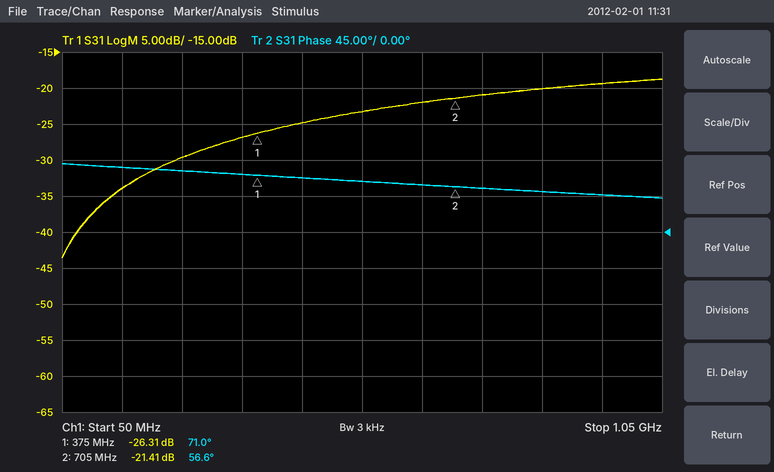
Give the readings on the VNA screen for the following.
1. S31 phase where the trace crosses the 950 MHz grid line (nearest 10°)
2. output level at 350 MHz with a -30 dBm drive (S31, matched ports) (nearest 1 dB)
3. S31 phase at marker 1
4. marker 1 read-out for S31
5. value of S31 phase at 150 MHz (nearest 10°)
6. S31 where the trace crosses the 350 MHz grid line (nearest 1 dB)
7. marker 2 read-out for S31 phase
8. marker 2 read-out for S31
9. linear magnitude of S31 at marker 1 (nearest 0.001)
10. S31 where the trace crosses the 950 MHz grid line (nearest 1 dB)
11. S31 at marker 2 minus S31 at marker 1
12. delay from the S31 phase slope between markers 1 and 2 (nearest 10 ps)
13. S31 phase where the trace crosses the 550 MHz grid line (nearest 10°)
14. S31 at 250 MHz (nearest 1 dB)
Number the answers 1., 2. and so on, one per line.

1. 50°
2. -57 dBm
3. 71.0°
4. -26.31 dB
5. 80°
6. -27 dB
7. 56.6°
8. -21.41 dB
9. 0.048
10. -19 dB
11. 4.90 dB
12. 120 ps
13. 60°
14. -30 dB
